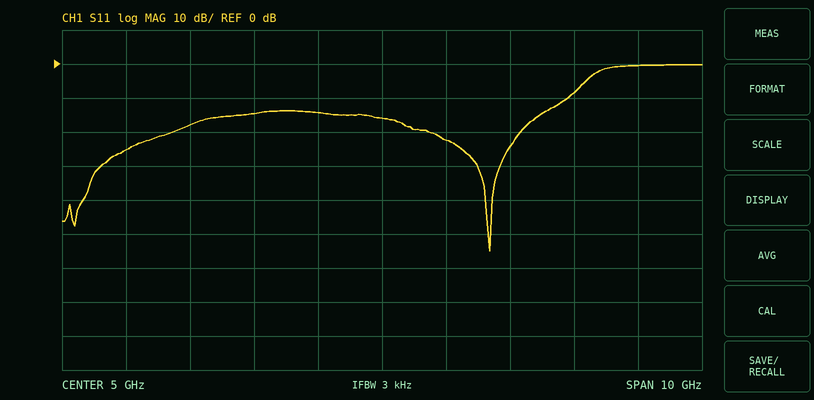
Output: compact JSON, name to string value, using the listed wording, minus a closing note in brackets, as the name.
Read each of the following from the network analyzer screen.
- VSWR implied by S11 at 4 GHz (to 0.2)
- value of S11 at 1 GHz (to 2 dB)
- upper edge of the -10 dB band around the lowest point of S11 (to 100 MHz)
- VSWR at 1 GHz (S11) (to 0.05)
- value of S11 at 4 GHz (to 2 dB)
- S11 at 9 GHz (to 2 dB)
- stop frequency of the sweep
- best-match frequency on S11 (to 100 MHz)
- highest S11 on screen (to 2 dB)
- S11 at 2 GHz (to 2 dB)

{"VSWR implied by S11 at 4 GHz": "1.4", "value of S11 at 1 GHz": "-26 dB", "upper edge of the -10 dB band around the lowest point of S11": "7.9 GHz", "VSWR at 1 GHz (S11)": "1.10", "value of S11 at 4 GHz": "-14 dB", "S11 at 9 GHz": "0 dB", "stop frequency of the sweep": "10 GHz", "best-match frequency on S11": "6.7 GHz", "highest S11 on screen": "0 dB", "S11 at 2 GHz": "-18 dB"}
